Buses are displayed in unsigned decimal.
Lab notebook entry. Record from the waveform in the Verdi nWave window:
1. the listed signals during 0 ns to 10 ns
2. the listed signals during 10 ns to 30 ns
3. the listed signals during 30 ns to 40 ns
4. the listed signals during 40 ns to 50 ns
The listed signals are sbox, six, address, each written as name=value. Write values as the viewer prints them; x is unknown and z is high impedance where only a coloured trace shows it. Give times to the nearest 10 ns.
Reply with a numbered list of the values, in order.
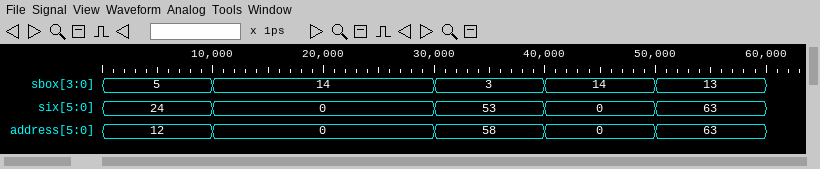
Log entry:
1. sbox=5, six=24, address=12
2. sbox=14, six=0, address=0
3. sbox=3, six=53, address=58
4. sbox=14, six=0, address=0
